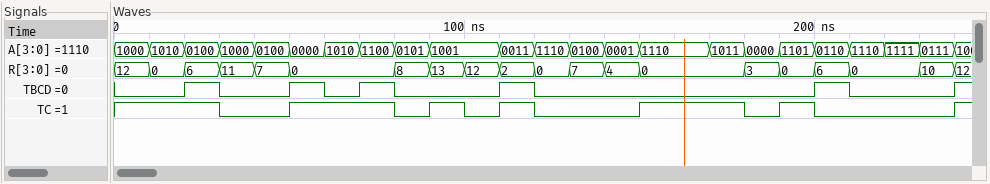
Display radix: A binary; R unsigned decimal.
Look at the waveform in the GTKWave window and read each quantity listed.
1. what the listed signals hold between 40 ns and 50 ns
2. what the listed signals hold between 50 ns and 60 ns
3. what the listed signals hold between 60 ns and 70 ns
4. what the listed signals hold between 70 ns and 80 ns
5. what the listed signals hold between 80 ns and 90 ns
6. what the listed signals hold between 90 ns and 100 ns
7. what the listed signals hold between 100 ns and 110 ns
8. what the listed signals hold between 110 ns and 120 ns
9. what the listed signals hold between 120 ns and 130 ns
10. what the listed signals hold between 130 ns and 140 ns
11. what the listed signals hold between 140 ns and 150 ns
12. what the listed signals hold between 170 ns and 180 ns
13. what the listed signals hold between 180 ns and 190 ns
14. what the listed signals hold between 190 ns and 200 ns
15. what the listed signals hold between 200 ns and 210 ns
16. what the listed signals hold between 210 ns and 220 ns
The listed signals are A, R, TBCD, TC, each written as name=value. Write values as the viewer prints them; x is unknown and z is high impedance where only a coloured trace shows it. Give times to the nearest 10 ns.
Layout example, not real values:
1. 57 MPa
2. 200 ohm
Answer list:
1. A=0100, R=7, TBCD=0, TC=0
2. A=0000, R=0, TBCD=1, TC=1
3. A=1010, R=0, TBCD=0, TC=1
4. A=1100, R=0, TBCD=1, TC=1
5. A=0101, R=8, TBCD=0, TC=0
6. A=1001, R=13, TBCD=0, TC=1
7. A=1001, R=12, TBCD=0, TC=0
8. A=0011, R=2, TBCD=1, TC=1
9. A=1110, R=0, TBCD=0, TC=0
10. A=0100, R=7, TBCD=0, TC=0
11. A=0001, R=4, TBCD=0, TC=0
12. A=1011, R=0, TBCD=0, TC=1
13. A=0000, R=3, TBCD=0, TC=0
14. A=1101, R=0, TBCD=0, TC=1
15. A=0110, R=6, TBCD=1, TC=0
16. A=1110, R=0, TBCD=0, TC=0
